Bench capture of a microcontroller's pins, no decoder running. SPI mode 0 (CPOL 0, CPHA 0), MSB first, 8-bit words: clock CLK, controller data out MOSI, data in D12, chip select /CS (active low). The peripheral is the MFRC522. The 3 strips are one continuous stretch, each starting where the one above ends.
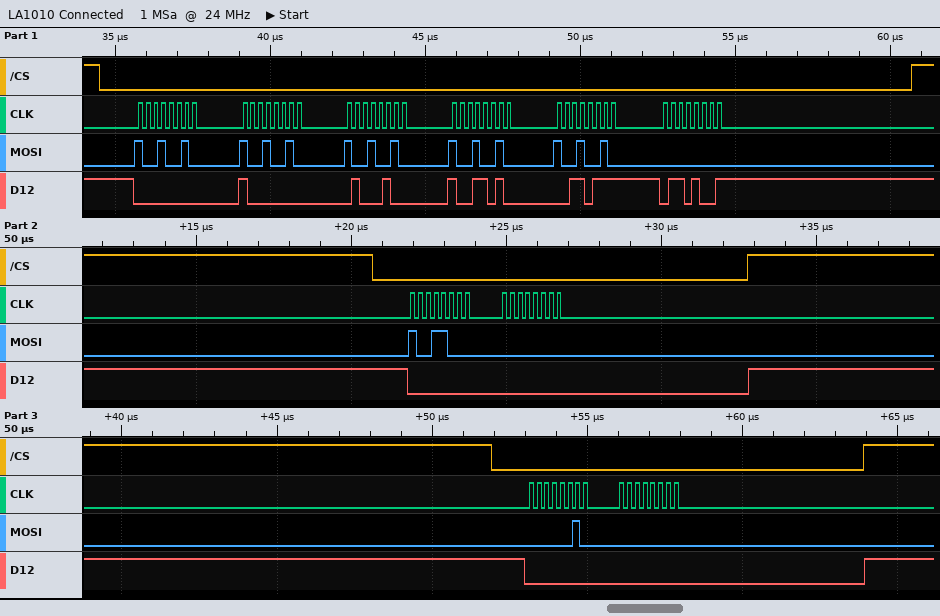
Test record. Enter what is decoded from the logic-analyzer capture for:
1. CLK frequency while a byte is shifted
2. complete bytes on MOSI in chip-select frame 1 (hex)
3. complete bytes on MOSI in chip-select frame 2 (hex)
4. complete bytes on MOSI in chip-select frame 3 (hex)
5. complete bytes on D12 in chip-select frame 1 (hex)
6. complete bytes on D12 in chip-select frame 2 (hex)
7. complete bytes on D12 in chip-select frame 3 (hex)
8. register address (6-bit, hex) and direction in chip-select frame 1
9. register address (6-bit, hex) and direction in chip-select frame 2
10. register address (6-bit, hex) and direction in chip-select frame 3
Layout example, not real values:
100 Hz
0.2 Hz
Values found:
4 MHz
92 92 92 92 92 00
98 00
02 00
00 80 44 9A 37 69
00 00
00 00
0x09 read
0x0C read
0x01 write
